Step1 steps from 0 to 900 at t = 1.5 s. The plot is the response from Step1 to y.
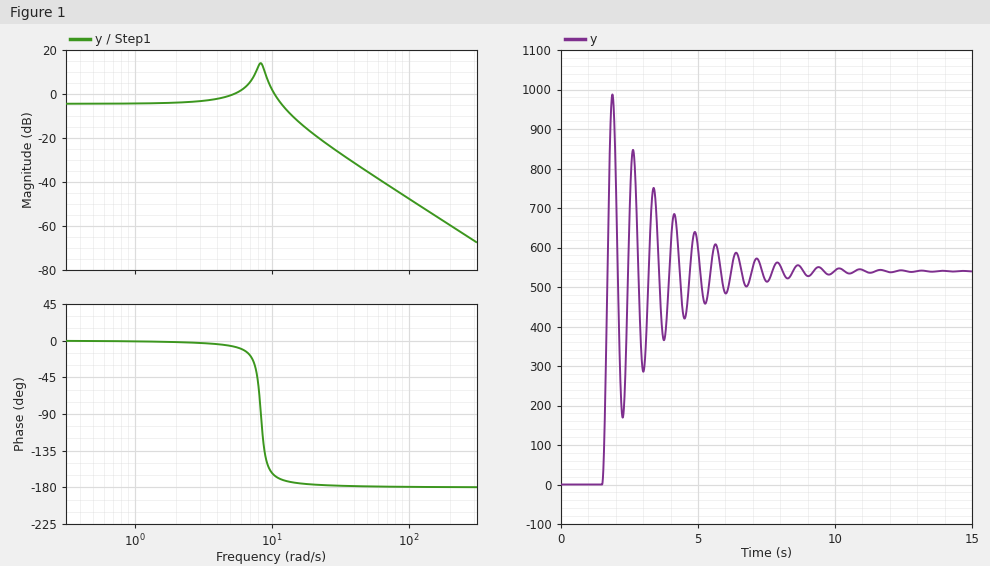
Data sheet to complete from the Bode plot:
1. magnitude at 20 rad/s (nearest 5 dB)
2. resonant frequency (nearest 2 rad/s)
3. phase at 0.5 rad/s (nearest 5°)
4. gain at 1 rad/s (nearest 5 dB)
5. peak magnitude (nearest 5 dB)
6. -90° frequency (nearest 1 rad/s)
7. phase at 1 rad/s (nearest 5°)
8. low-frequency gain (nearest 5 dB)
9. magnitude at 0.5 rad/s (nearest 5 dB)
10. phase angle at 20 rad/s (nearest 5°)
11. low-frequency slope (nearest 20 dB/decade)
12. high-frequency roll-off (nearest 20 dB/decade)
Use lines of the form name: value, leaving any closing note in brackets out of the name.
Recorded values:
magnitude at 20 rad/s: -20 dB
resonant frequency: 8 rad/s
phase at 0.5 rad/s: 0°
gain at 1 rad/s: -5 dB
peak magnitude: 15 dB
-90° frequency: 8 rad/s
phase at 1 rad/s: 0°
low-frequency gain: -5 dB
magnitude at 0.5 rad/s: -5 dB
phase angle at 20 rad/s: -175°
low-frequency slope: 0 dB/decade
high-frequency roll-off: -40 dB/decade
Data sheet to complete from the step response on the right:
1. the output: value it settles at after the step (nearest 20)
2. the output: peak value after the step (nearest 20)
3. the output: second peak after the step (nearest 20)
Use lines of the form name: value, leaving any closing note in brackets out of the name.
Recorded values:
the output: value it settles at after the step: 540
the output: peak value after the step: 980
the output: second peak after the step: 840
